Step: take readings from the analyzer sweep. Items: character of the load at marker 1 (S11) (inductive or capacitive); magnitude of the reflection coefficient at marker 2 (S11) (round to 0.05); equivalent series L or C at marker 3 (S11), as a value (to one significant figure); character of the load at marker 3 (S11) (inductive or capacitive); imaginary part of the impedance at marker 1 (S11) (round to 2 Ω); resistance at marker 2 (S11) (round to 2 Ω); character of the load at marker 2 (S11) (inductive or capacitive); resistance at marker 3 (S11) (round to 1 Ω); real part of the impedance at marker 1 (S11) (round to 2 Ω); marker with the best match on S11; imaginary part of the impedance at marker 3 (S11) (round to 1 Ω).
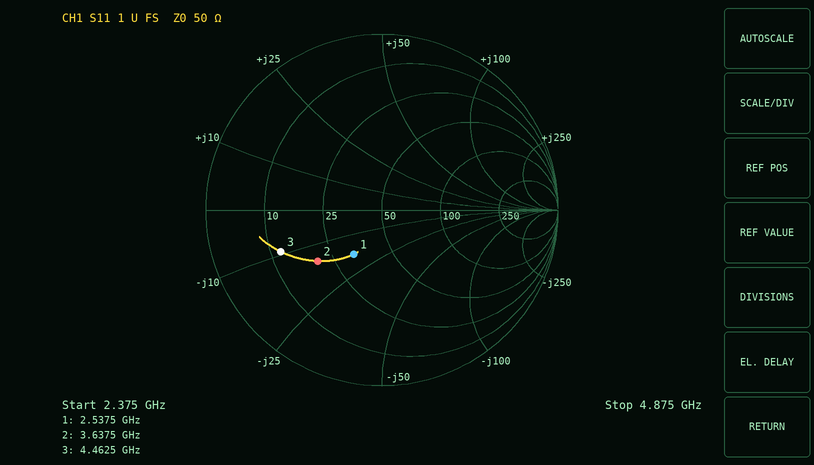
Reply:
capacitive
0.45
4 pF
capacitive
-18 Ω
20 Ω
capacitive
12 Ω
32 Ω
marker 1
-9 Ω
